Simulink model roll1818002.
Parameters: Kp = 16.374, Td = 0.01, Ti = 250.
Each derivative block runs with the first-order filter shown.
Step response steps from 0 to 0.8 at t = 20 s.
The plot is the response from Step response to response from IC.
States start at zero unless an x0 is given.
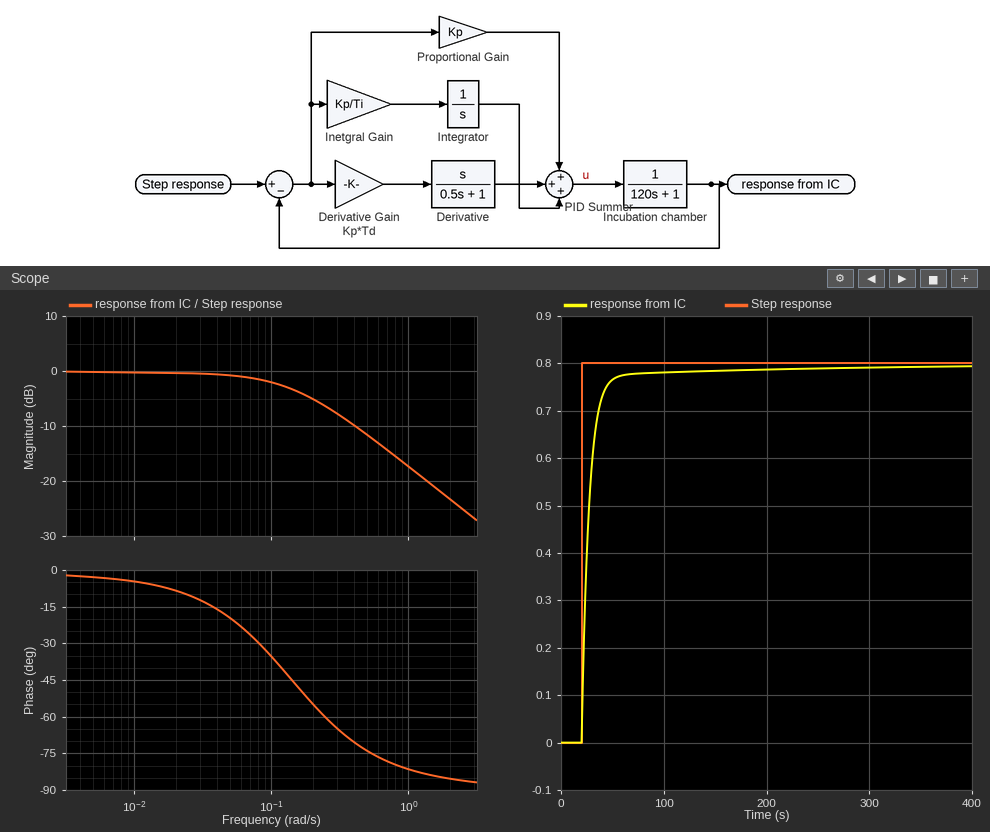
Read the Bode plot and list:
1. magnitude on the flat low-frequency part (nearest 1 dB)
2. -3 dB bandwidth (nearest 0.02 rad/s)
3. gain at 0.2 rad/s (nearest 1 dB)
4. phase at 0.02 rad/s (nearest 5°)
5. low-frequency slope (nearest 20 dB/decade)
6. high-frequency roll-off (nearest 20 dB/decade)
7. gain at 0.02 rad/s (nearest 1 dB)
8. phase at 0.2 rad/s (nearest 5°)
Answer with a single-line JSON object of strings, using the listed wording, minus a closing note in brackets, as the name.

{"magnitude on the flat low-frequency part": "0 dB", "-3 dB bandwidth": "0.14 rad/s", "gain at 0.2 rad/s": "-5 dB", "phase at 0.02 rad/s": "-10°", "low-frequency slope": "0 dB/decade", "high-frequency roll-off": "-20 dB/decade", "gain at 0.02 rad/s": "0 dB", "phase at 0.2 rad/s": "-55°"}
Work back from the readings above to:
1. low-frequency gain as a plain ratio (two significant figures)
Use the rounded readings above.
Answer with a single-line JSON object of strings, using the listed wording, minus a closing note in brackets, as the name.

{"low-frequency gain as a plain ratio": "1.0"}
